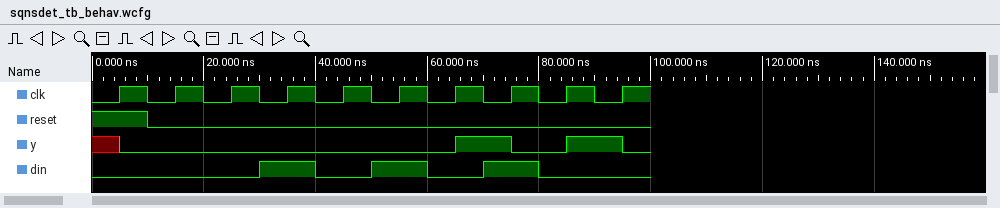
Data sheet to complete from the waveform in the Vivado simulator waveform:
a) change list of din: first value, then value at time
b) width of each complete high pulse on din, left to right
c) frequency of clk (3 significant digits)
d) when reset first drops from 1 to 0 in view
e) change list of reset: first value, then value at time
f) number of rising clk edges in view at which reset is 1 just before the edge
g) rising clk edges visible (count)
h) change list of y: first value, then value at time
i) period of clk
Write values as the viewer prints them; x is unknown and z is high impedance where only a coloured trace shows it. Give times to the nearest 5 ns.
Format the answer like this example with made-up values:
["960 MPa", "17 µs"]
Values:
["0, 1 at 30 ns, 0 at 40 ns, 1 at 50 ns, 0 at 60 ns, 1 at 70 ns, 0 at 80 ns", "10 ns, 10 ns, 10 ns", "100 MHz", "10 ns", "1, 0 at 10 ns", "1", "10", "x, 0 at 5 ns, 1 at 65 ns, 0 at 75 ns, 1 at 85 ns, 0 at 95 ns", "10 ns"]
